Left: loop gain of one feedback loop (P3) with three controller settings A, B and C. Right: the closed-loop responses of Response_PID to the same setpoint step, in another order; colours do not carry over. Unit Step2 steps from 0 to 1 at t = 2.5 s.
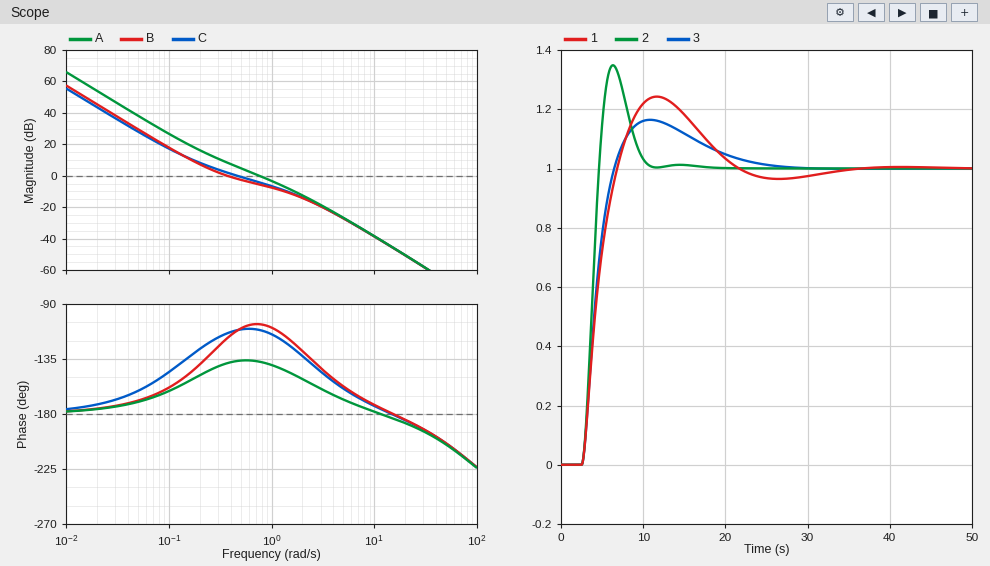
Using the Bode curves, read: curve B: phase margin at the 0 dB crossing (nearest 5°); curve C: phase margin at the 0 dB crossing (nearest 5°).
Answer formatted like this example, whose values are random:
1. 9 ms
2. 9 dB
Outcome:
1. 60°
2. 70°
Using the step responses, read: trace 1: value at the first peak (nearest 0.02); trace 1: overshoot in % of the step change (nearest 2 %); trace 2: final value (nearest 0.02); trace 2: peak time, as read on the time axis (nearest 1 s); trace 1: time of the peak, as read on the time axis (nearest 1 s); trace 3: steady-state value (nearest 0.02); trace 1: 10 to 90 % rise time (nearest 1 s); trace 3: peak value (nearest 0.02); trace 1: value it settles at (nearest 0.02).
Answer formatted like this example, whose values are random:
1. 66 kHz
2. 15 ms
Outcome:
1. 1.24
2. 24 %
3. 1.00
4. 6 s
5. 12 s
6. 1.00
7. 3 s
8. 1.16
9. 1.00
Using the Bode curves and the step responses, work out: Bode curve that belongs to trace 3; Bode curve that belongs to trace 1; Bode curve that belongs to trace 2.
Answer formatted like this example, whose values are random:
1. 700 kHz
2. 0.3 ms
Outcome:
1. C
2. B
3. A
